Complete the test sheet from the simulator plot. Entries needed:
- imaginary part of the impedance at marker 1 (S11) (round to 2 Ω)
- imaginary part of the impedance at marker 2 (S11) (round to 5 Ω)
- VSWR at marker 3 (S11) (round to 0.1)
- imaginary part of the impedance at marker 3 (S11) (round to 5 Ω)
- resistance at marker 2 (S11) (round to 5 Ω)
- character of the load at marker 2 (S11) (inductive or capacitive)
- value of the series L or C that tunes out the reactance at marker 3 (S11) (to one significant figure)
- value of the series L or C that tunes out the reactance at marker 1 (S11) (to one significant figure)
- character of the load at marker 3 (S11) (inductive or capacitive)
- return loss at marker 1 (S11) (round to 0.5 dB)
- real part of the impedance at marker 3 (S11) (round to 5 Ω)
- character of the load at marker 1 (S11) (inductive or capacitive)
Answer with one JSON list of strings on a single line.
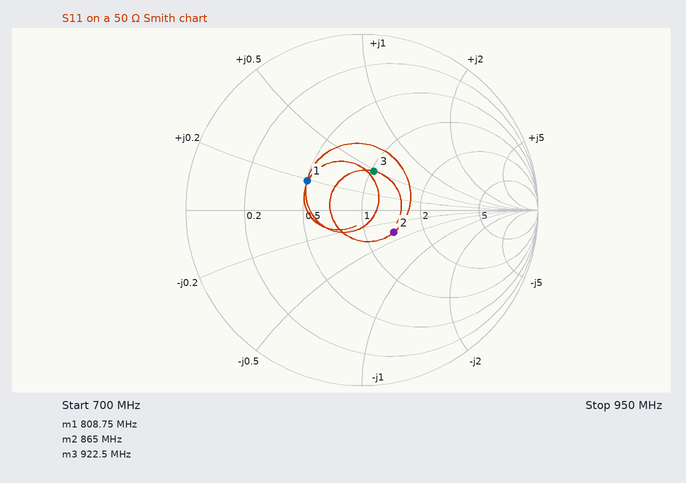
["+10 Ω", "-20 Ω", "1.6", "+25 Ω", "70 Ω", "capacitive", "7 pF", "20 pF", "inductive", "9.0 dB", "50 Ω", "inductive"]
